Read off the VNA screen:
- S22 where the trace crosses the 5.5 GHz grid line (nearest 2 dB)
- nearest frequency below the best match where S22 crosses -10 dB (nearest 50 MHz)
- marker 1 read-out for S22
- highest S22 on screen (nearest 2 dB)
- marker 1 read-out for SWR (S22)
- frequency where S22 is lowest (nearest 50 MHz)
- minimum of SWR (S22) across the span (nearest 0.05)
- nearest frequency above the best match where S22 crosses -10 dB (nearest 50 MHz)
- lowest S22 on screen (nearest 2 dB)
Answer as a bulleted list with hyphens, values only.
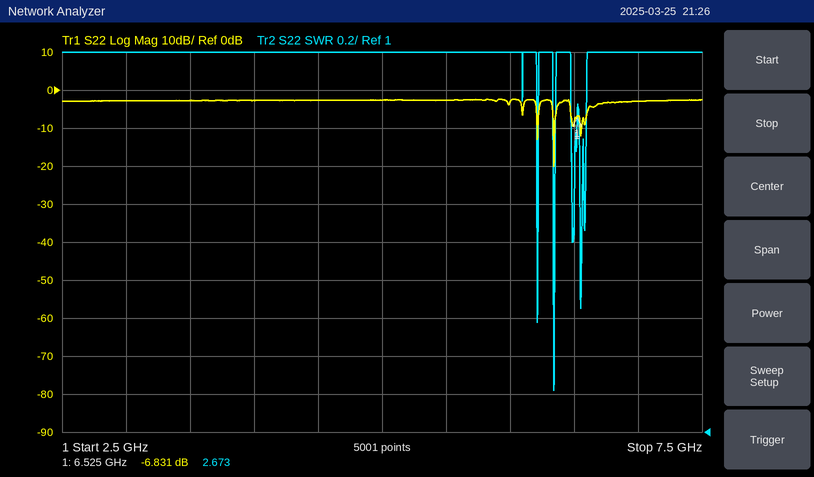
- -2 dB
- 6.35 GHz
- -6.831 dB
- -2 dB
- 2.673
- 6.35 GHz
- 1.20
- 6.35 GHz
- -20 dB
